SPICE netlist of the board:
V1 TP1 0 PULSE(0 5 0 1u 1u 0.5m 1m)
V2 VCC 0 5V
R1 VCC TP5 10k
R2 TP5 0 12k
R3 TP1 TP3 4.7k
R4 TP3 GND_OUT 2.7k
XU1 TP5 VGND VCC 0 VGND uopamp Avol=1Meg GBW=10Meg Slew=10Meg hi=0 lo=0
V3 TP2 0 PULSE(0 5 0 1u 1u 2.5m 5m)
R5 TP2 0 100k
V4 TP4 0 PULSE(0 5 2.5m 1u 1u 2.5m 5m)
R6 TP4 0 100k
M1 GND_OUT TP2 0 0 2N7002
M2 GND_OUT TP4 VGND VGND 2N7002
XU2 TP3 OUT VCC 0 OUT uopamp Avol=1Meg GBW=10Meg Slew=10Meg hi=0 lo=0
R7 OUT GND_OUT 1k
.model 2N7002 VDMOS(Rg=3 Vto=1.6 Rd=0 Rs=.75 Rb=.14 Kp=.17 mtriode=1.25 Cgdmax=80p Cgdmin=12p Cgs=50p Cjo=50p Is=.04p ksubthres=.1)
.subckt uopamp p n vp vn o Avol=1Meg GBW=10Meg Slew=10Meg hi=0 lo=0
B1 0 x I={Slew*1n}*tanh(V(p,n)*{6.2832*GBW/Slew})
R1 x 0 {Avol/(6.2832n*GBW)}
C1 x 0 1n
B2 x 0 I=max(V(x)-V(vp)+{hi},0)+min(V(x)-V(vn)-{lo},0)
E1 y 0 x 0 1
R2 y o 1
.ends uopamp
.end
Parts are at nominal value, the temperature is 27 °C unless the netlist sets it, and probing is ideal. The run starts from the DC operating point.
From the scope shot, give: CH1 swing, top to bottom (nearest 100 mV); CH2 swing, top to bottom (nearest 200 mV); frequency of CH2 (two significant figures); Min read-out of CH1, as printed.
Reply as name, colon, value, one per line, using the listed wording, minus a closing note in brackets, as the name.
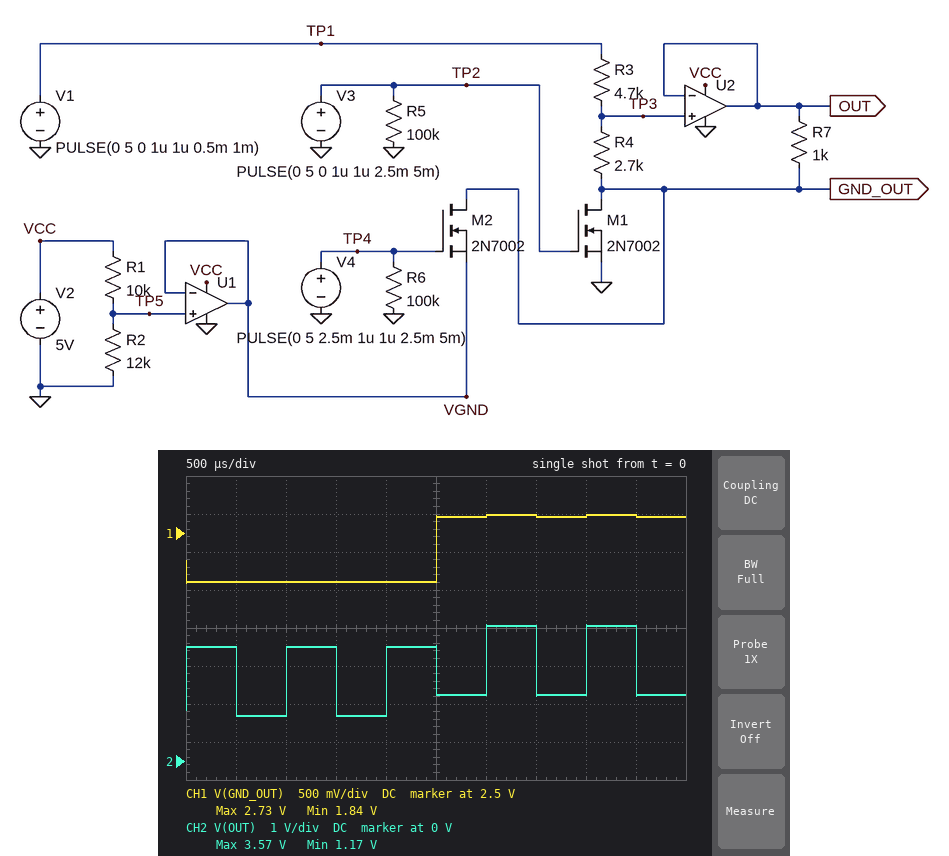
CH1 swing, top to bottom: 900 mV
CH2 swing, top to bottom: 2.4 V
frequency of CH2: 1.0 kHz
Min read-out of CH1, as printed: 1.84 V
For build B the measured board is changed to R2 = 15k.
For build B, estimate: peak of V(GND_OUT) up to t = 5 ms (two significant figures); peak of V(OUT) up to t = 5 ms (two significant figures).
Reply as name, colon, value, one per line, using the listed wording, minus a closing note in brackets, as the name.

peak of V(GND_OUT) up to t = 5 ms: 3.0 V
peak of V(OUT) up to t = 5 ms: 3.7 V
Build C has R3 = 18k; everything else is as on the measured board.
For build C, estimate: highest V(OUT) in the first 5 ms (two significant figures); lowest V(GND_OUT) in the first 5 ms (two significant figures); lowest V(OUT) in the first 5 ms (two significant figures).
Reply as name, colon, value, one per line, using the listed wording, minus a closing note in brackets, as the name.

highest V(OUT) in the first 5 ms: 3.0 V
lowest V(GND_OUT) in the first 5 ms: 1.8 V
lowest V(OUT) in the first 5 ms: 1.6 V
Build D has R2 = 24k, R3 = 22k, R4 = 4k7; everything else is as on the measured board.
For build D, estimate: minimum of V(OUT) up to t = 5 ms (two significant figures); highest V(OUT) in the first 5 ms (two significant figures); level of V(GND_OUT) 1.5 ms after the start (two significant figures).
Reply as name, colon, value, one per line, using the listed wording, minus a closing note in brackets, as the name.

minimum of V(OUT) up to t = 5 ms: 2.2 V
highest V(OUT) in the first 5 ms: 4.8 V
level of V(GND_OUT) 1.5 ms after the start: 2.6 V
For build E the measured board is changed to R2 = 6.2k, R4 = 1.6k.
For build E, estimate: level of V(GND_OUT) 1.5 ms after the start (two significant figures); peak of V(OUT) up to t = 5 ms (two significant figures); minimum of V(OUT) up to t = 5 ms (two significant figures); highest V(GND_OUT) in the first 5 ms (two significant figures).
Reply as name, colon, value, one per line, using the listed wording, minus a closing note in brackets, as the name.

level of V(GND_OUT) 1.5 ms after the start: 1.1 V
peak of V(OUT) up to t = 5 ms: 2.7 V
minimum of V(OUT) up to t = 5 ms: 800 mV
highest V(GND_OUT) in the first 5 ms: 1.9 V
